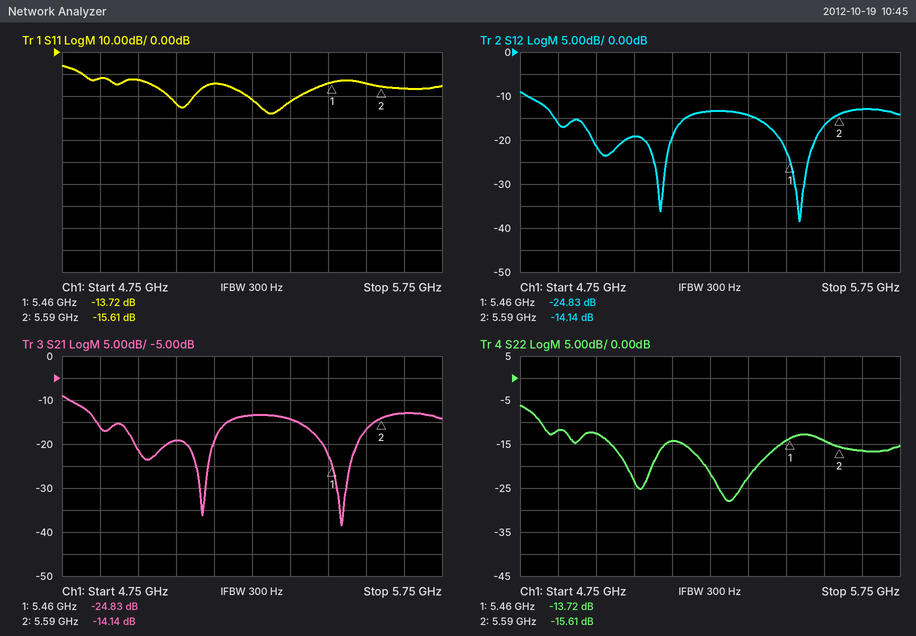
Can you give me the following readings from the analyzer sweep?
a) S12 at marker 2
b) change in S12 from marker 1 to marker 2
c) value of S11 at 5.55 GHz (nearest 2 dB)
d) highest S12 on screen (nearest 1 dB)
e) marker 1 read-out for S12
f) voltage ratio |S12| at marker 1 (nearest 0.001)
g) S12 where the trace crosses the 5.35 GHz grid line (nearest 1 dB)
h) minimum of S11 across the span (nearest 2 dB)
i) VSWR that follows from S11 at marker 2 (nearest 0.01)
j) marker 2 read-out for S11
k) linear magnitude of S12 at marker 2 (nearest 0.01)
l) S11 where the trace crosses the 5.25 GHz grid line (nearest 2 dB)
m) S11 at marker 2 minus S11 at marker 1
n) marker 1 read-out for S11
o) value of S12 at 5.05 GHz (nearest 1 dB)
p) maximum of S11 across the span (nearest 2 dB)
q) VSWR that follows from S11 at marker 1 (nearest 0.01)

-14.14 dB
10.69 dB
-14 dB
-9 dB
-24.83 dB
0.057
-14 dB
-28 dB
1.40
-15.61 dB
0.20
-22 dB
-1.89 dB
-13.72 dB
-19 dB
-6 dB
1.52
